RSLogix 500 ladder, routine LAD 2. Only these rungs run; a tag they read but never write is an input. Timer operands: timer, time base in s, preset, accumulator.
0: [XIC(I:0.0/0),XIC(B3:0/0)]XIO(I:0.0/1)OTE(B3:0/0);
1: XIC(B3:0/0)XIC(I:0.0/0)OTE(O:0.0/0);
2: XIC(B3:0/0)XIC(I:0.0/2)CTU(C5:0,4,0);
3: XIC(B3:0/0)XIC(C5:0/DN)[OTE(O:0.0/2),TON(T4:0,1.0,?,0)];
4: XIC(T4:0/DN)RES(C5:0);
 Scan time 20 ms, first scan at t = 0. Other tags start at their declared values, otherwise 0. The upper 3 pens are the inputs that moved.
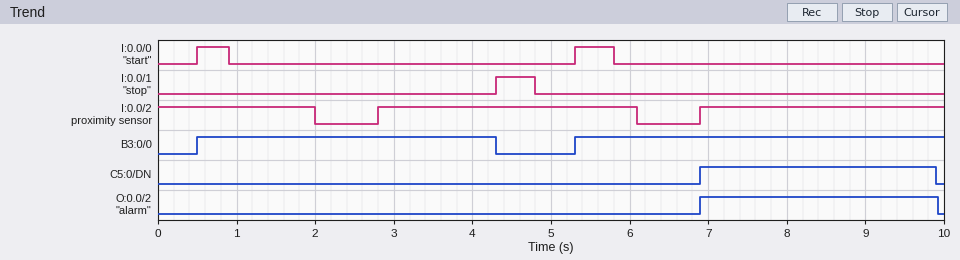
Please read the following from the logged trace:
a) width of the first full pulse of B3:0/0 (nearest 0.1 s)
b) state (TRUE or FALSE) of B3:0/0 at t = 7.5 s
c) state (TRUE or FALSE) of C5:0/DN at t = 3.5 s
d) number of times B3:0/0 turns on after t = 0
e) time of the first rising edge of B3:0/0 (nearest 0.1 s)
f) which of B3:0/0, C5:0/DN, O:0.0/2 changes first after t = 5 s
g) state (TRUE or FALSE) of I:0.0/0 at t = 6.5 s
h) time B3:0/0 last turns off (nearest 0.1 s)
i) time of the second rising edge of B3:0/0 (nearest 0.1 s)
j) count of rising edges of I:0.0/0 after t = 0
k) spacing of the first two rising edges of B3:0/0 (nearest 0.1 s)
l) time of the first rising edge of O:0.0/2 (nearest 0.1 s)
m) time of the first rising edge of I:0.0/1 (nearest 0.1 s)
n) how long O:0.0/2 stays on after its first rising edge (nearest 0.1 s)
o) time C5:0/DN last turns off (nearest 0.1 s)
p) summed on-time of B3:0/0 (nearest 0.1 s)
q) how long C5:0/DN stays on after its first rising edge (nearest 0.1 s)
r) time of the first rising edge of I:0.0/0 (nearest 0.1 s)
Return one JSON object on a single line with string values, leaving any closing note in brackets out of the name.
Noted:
{"width of the first full pulse of B3:0/0": "3.8 s", "state (TRUE or FALSE) of B3:0/0 at t = 7.5 s": "TRUE", "state (TRUE or FALSE) of C5:0/DN at t = 3.5 s": "FALSE", "number of times B3:0/0 turns on after t = 0": "2", "time of the first rising edge of B3:0/0": "0.5 s", "which of B3:0/0, C5:0/DN, O:0.0/2 changes first after t = 5 s": "B3:0/0", "state (TRUE or FALSE) of I:0.0/0 at t = 6.5 s": "FALSE", "time B3:0/0 last turns off": "4.3 s", "time of the second rising edge of B3:0/0": "5.3 s", "count of rising edges of I:0.0/0 after t = 0": "2", "spacing of the first two rising edges of B3:0/0": "4.8 s", "time of the first rising edge of O:0.0/2": "6.9 s", "time of the first rising edge of I:0.0/1": "4.3 s", "how long O:0.0/2 stays on after its first rising edge": "3.0 s", "time C5:0/DN last turns off": "9.9 s", "summed on-time of B3:0/0": "8.5 s", "how long C5:0/DN stays on after its first rising edge": "3.0 s", "time of the first rising edge of I:0.0/0": "0.5 s"}
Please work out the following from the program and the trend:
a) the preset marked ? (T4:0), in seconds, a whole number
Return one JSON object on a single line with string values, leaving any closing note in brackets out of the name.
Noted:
{"the preset marked ? (T4:0), in seconds, a whole number": "3 s"}
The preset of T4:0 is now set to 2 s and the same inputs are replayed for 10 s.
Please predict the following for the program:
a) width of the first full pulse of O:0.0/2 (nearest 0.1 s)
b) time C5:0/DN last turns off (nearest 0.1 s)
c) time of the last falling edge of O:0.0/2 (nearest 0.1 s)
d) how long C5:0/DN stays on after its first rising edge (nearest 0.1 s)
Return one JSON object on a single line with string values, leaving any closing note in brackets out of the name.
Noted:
{"width of the first full pulse of O:0.0/2": "2.0 s", "time C5:0/DN last turns off": "8.9 s", "time of the last falling edge of O:0.0/2": "8.9 s", "how long C5:0/DN stays on after its first rising edge": "2.0 s"}
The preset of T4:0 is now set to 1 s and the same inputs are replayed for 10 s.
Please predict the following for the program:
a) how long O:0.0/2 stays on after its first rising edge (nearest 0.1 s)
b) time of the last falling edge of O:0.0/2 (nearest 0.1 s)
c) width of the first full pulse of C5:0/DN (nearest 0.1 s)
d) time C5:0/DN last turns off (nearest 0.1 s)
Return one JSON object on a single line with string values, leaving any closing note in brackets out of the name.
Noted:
{"how long O:0.0/2 stays on after its first rising edge": "1.0 s", "time of the last falling edge of O:0.0/2": "7.9 s", "width of the first full pulse of C5:0/DN": "1.0 s", "time C5:0/DN last turns off": "7.9 s"}
